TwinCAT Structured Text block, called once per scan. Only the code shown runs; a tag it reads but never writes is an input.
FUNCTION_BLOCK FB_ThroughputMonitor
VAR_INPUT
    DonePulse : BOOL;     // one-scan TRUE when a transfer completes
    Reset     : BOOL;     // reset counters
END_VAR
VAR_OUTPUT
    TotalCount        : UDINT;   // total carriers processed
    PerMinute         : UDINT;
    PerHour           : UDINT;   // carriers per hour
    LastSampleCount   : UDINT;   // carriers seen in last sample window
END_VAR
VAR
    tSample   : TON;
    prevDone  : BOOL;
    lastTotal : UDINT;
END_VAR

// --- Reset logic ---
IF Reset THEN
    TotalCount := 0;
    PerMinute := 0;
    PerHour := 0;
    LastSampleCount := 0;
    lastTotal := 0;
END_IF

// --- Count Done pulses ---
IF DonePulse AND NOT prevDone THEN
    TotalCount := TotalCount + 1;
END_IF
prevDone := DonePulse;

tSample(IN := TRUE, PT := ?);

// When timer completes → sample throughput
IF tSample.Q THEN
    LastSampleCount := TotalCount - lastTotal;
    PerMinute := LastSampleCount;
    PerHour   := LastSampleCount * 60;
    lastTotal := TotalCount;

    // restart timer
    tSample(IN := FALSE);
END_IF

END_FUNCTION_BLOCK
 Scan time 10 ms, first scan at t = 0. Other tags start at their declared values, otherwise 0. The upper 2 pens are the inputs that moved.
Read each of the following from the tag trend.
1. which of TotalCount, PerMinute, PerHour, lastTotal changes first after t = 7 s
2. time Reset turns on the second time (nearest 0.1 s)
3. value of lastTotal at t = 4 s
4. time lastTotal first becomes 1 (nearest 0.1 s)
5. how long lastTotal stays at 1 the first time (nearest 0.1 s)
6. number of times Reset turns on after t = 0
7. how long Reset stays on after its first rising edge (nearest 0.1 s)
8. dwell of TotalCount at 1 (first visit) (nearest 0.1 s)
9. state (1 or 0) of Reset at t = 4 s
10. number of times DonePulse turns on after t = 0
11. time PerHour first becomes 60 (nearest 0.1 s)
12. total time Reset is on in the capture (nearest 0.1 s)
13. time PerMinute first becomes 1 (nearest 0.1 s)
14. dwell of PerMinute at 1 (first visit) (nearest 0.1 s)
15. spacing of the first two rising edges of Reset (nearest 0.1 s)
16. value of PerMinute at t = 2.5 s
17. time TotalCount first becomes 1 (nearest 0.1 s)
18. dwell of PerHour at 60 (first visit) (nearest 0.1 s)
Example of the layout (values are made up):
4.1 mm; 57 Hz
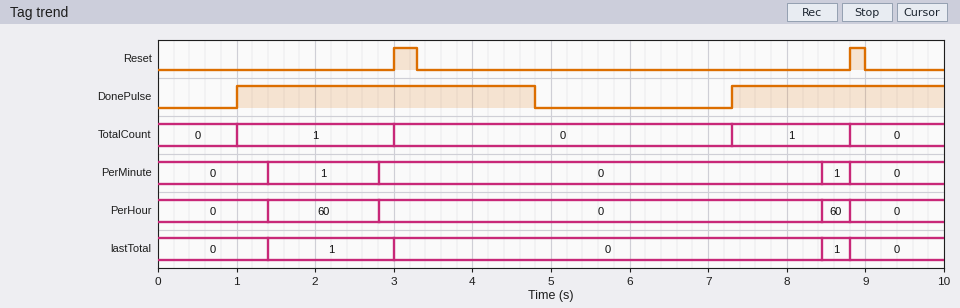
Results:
TotalCount; 8.8 s; 0; 1.4 s; 1.6 s; 2; 0.3 s; 2.0 s; 0; 2; 1.4 s; 0.5 s; 1.4 s; 1.4 s; 5.8 s; 1; 1.0 s; 1.4 s
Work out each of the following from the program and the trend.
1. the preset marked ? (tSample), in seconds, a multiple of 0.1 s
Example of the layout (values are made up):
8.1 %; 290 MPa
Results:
1.4 s
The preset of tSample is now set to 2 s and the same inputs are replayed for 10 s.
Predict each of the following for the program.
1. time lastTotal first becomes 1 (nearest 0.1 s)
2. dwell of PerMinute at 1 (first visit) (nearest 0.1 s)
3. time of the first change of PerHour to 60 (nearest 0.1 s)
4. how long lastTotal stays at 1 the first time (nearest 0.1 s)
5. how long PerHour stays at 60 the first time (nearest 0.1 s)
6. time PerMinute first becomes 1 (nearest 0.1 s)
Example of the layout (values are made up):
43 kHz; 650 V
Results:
2.0 s; 1.0 s; 2.0 s; 1.0 s; 1.0 s; 2.0 s
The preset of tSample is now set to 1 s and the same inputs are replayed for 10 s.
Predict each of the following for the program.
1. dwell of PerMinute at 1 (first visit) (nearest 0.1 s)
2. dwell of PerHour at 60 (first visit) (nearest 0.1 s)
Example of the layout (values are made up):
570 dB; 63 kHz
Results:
1.0 s; 1.0 s
